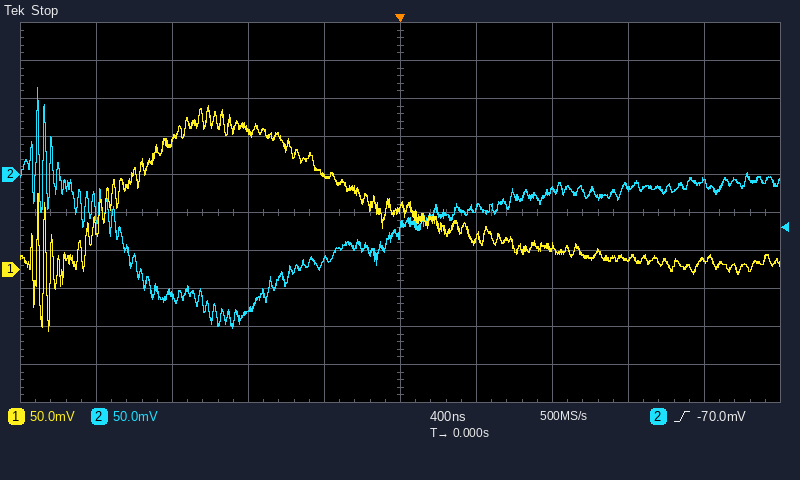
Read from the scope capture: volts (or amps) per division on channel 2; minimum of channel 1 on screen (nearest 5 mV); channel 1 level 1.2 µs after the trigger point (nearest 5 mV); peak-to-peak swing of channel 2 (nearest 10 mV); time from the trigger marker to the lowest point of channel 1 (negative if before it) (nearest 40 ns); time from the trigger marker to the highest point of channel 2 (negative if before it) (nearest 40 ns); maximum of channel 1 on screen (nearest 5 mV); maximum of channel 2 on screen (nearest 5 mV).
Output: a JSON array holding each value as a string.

["50 mV", "-80 mV", "15 mV", "320 mV", "-1.84 µs", "-1.92 µs", "215 mV", "115 mV"]
